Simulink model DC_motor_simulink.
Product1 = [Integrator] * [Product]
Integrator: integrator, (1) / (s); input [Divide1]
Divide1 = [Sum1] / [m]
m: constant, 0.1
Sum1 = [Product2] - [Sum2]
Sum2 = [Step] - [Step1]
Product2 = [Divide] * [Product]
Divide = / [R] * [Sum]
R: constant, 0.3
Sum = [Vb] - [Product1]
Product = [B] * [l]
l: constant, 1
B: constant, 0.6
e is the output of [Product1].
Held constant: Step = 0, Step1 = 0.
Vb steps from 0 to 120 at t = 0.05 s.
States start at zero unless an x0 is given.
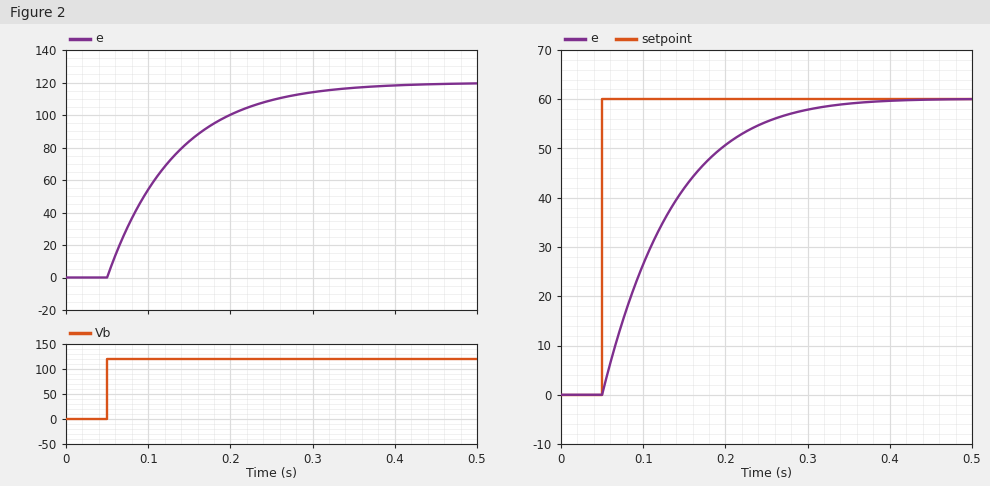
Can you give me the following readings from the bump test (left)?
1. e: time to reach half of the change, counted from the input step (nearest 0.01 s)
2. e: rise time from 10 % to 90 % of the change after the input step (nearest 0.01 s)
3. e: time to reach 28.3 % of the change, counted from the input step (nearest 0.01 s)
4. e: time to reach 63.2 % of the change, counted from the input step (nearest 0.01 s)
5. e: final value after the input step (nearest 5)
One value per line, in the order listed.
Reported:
0.06 s
0.18 s
0.03 s
0.08 s
120
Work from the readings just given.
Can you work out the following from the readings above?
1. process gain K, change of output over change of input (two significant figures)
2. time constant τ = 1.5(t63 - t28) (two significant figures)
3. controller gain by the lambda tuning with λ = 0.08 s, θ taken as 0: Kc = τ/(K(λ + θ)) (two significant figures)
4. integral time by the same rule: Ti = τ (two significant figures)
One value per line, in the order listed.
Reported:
1.0
0.075 s
0.94
0.075 s
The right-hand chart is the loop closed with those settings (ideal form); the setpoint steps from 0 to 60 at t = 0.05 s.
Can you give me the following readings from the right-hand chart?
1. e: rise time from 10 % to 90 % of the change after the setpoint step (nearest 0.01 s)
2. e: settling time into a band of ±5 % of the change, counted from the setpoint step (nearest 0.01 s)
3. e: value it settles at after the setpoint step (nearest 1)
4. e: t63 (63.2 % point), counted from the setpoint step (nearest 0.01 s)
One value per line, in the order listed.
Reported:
0.17 s
0.23 s
60
0.08 s
